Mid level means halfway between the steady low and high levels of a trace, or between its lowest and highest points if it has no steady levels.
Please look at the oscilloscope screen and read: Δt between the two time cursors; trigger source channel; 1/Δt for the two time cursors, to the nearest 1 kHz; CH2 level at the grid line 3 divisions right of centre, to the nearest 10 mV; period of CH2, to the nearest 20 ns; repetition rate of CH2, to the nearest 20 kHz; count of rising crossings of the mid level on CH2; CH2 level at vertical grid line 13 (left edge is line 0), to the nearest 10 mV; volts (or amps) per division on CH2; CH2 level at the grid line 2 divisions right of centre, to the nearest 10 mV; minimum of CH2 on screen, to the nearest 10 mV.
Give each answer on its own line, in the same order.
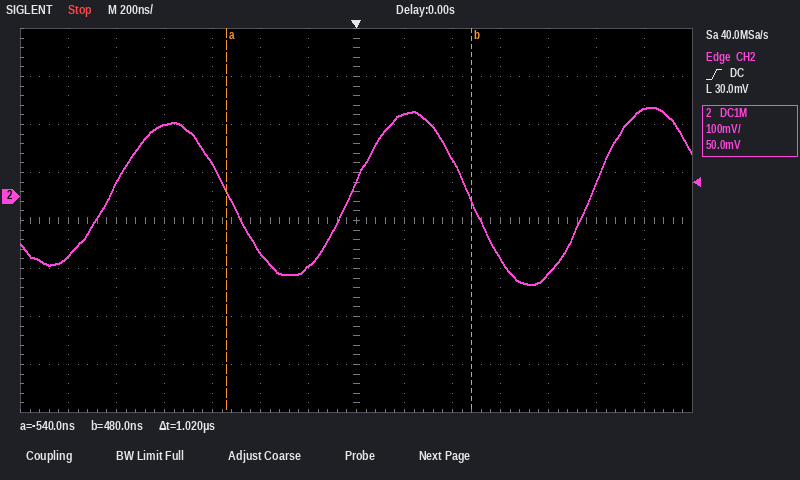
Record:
1.02 µs
CH2
980 kHz
-130 mV
1.00 µs
1.00 MHz
3
180 mV
100 mV
80 mV
-180 mV
